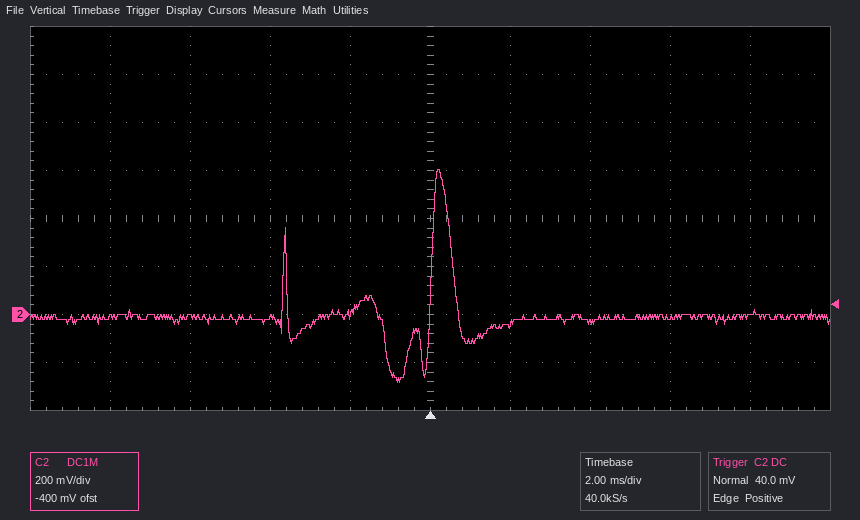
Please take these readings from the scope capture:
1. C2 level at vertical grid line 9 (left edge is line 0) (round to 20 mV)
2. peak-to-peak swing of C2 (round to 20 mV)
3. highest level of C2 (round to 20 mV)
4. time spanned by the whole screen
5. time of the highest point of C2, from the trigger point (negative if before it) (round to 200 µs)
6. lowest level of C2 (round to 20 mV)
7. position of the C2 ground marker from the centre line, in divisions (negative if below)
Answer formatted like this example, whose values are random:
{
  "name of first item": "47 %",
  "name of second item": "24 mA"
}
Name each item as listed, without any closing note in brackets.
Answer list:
{
  "C2 level at vertical grid line 9 (left edge is line 0)": "0 mV",
  "peak-to-peak swing of C2": "880 mV",
  "highest level of C2": "600 mV",
  "time spanned by the whole screen": "20 ms",
  "time of the highest point of C2, from the trigger point (negative if before it)": "+200 µs",
  "lowest level of C2": "-280 mV",
  "position of the C2 ground marker from the centre line, in divisions": "-2.0 div"
}
